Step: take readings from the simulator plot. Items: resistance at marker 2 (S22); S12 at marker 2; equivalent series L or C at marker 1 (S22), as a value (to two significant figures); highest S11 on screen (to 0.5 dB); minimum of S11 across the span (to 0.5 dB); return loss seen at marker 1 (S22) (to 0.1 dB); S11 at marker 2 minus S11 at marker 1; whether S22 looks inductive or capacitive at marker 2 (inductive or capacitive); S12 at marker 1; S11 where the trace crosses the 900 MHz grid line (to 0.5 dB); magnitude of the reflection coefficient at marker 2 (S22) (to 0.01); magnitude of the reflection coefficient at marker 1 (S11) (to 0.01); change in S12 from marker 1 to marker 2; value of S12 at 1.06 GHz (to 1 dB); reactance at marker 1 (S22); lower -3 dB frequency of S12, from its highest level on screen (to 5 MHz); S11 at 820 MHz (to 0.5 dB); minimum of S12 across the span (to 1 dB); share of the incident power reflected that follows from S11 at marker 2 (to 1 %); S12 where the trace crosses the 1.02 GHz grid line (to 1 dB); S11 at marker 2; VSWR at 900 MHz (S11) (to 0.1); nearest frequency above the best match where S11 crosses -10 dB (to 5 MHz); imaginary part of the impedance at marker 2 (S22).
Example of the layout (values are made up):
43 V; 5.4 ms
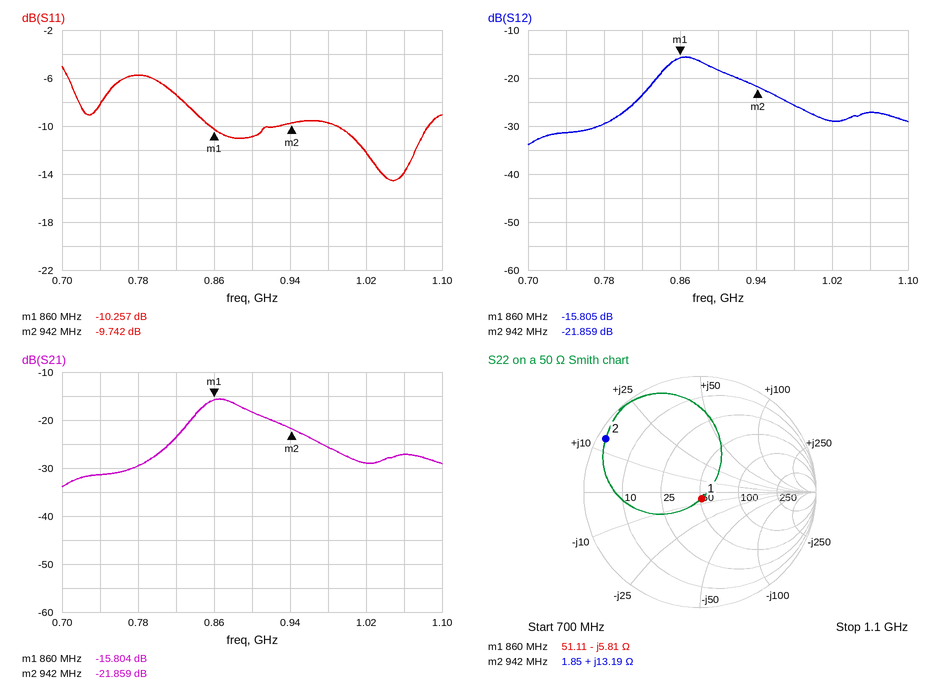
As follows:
1.85 Ω; -21.859 dB; 32 pF; -5.0 dB; -14.5 dB; 24.7 dB; 0.515 dB; inductive; -15.805 dB; -11.0 dB; 0.93; 0.31; -6.054 dB; -27 dB; -5.81 Ω; 840 MHz; -7.5 dB; -34 dB; 11 %; -29 dB; -9.742 dB; 1.8; 1.085 GHz; +13.19 Ω
